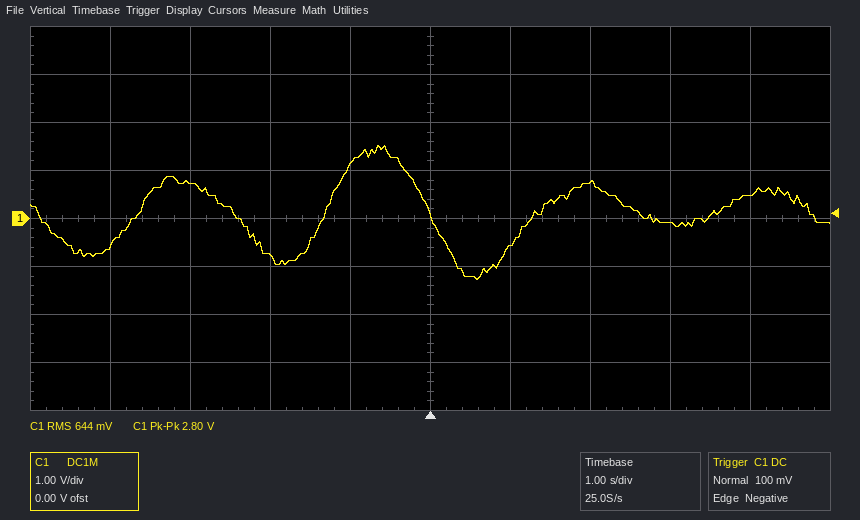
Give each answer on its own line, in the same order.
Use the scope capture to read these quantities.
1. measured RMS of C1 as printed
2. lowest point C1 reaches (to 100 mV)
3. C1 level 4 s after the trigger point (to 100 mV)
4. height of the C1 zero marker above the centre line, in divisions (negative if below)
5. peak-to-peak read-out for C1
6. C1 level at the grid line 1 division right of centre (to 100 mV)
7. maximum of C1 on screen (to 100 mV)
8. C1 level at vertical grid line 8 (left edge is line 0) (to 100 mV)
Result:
644 mV
-1.3 V
500 mV
0.0 div
2.80 V
-600 mV
1.5 V
-100 mV
